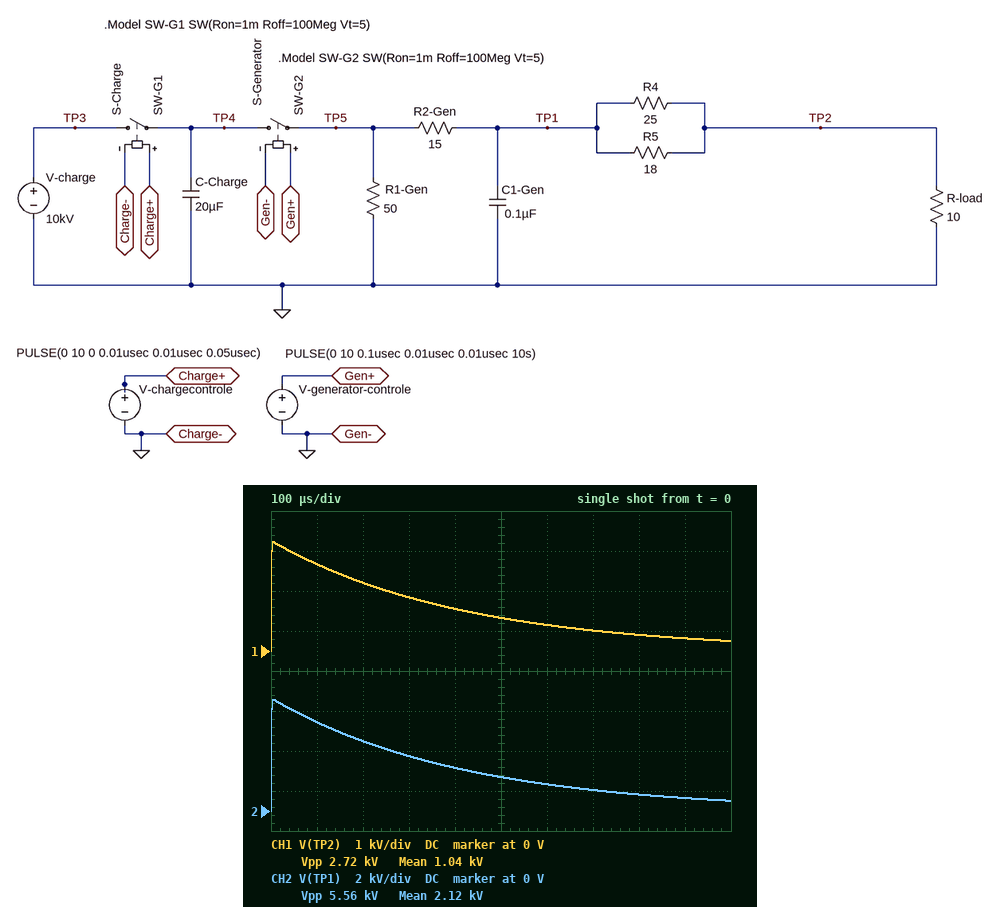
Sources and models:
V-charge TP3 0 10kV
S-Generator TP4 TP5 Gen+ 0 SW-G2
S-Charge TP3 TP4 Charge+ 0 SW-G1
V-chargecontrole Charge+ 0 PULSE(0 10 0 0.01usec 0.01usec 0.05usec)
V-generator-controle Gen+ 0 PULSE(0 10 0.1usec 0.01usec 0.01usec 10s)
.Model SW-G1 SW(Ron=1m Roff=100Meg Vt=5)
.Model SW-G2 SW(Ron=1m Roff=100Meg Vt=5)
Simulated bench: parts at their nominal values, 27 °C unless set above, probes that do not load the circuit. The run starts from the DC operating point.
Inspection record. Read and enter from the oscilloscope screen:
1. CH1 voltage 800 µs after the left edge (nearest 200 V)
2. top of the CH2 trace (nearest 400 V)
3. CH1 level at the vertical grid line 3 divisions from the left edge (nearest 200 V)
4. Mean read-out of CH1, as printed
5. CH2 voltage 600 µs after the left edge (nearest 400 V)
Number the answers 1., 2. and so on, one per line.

1. 400 V
2. 5.6 kV
3. 1.4 kV
4. 1.04 kV
5. 1.2 kV
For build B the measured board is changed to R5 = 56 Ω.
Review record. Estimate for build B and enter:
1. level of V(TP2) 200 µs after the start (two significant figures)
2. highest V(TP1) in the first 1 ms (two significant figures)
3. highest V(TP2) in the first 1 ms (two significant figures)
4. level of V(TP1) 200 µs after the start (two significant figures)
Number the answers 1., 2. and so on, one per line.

1. 1.5 kV
2. 6.2 kV
3. 2.3 kV
4. 4.1 kV
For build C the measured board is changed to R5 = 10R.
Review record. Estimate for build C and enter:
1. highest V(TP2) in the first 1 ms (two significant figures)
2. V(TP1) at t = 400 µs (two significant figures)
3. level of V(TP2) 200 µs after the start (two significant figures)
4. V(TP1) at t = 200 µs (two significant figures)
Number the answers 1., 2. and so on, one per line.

1. 3.0 kV
2. 1.9 kV
3. 1.8 kV
4. 3.1 kV
